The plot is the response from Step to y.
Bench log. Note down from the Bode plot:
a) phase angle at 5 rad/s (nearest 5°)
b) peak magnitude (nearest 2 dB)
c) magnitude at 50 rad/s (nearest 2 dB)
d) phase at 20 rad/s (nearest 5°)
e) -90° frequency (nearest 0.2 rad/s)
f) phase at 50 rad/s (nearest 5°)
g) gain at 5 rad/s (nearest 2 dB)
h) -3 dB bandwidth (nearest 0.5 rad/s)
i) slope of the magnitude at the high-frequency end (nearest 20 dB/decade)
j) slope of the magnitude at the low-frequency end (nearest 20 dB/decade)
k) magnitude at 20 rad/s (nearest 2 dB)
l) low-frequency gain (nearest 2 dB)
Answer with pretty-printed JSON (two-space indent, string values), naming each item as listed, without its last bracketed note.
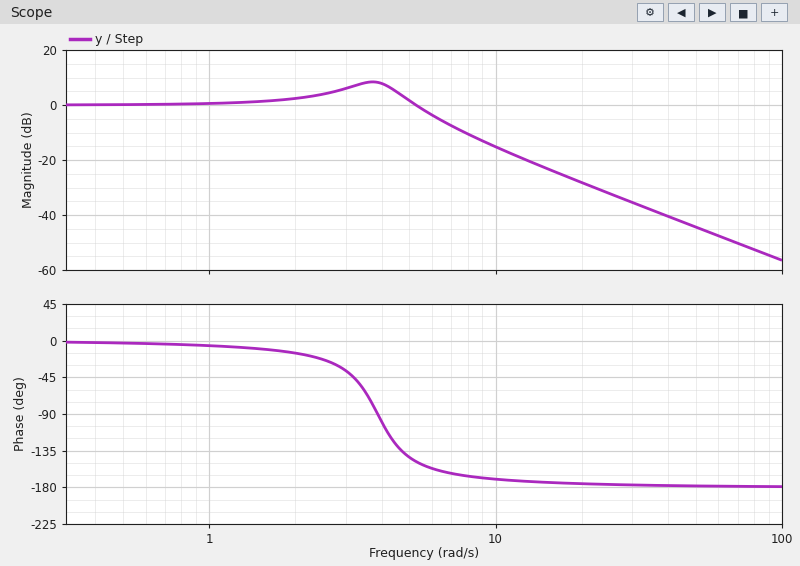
{
  "phase angle at 5 rad/s": "-145°",
  "peak magnitude": "8 dB",
  "magnitude at 50 rad/s": "-44 dB",
  "phase at 20 rad/s": "-175°",
  "-90° frequency": "3.8 rad/s",
  "phase at 50 rad/s": "-180°",
  "gain at 5 rad/s": "2 dB",
  "-3 dB bandwidth": "6.0 rad/s",
  "slope of the magnitude at the high-frequency end": "-40 dB/decade",
  "slope of the magnitude at the low-frequency end": "0 dB/decade",
  "magnitude at 20 rad/s": "-28 dB",
  "low-frequency gain": "0 dB"
}
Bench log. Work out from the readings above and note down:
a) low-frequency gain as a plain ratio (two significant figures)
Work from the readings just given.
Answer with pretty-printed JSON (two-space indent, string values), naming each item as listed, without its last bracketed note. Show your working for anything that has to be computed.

{
  "low-frequency gain as a plain ratio": "10^(0 / 20) = 1.0"
}
